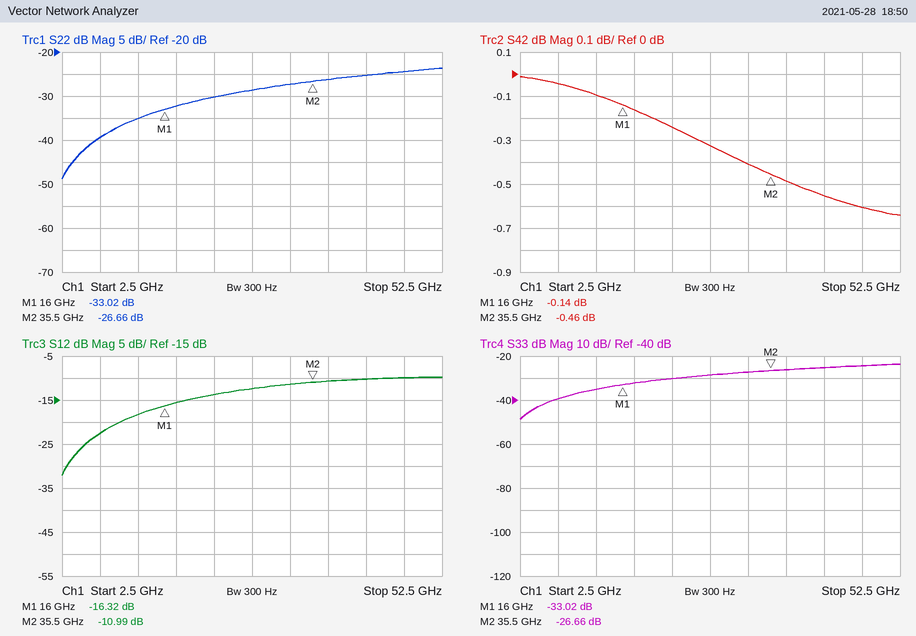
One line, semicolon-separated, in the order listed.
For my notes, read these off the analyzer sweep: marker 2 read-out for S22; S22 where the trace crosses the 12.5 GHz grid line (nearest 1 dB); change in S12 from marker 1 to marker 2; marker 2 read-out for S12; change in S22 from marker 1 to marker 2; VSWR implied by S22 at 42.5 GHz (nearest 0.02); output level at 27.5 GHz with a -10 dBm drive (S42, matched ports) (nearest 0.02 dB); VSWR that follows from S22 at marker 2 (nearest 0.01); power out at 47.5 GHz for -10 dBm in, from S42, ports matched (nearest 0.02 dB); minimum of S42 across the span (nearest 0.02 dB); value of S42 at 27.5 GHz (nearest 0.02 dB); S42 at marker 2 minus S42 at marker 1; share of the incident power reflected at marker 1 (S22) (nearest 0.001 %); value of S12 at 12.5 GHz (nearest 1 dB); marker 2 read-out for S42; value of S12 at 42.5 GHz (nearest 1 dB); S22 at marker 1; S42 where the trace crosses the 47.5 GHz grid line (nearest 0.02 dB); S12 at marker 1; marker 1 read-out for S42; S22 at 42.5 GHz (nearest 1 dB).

-26.66 dB; -35 dB; 5.33 dB; -10.99 dB; 6.36 dB; 1.12; -10.32 dBm; 1.10; -10.60 dBm; -0.64 dB; -0.32 dB; -0.32 dB; 0.050 %; -18 dB; -0.46 dB; -10 dB; -33.02 dB; -0.60 dB; -16.32 dB; -0.14 dB; -25 dB
